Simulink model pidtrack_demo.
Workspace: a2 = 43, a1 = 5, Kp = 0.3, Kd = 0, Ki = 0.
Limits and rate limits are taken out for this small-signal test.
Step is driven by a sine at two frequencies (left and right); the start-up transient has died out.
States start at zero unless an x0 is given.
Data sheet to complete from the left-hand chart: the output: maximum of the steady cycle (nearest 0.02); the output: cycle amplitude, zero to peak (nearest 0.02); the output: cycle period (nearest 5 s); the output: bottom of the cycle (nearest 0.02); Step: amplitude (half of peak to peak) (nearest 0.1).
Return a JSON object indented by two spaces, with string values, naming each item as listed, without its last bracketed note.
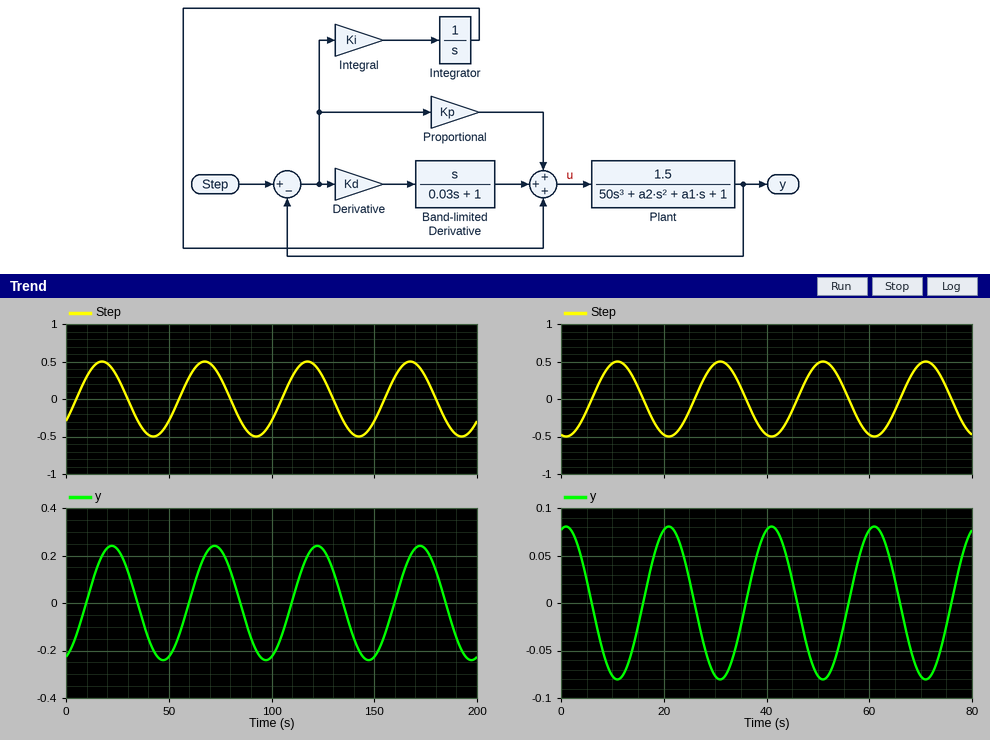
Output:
{
  "the output: maximum of the steady cycle": "0.24",
  "the output: cycle amplitude, zero to peak": "0.24",
  "the output: cycle period": "50 s",
  "the output: bottom of the cycle": "-0.24",
  "Step: amplitude (half of peak to peak)": "0.5"
}
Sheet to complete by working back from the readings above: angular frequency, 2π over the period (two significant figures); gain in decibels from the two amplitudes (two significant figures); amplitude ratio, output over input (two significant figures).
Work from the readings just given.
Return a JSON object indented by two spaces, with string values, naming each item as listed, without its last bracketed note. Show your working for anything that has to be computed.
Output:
{
  "angular frequency, 2π over the period": "2π / 50 = 0.13 rad/s",
  "gain in decibels from the two amplitudes": "20 log10(0.24 / 0.5) = -6.4 dB",
  "amplitude ratio, output over input": "0.24 / 0.5 = 0.48"
}
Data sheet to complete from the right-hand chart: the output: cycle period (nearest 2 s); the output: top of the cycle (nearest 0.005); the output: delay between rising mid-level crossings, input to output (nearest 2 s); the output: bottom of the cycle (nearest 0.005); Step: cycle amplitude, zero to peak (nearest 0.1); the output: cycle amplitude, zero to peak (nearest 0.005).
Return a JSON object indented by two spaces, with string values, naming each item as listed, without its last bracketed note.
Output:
{
  "the output: cycle period": "20 s",
  "the output: top of the cycle": "0.080",
  "the output: delay between rising mid-level crossings, input to output": "10 s",
  "the output: bottom of the cycle": "-0.080",
  "Step: cycle amplitude, zero to peak": "0.5",
  "the output: cycle amplitude, zero to peak": "0.080"
}
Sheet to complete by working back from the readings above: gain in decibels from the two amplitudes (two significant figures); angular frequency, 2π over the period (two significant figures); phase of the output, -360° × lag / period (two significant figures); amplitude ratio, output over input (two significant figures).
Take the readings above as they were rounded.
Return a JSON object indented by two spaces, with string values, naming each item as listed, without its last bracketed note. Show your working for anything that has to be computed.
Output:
{
  "gain in decibels from the two amplitudes": "20 log10(0.08 / 0.5) = -16 dB",
  "angular frequency, 2π over the period": "2π / 20 = 0.31 rad/s",
  "phase of the output, -360° × lag / period": "-360 × 10 / 20 = -180°",
  "amplitude ratio, output over input": "0.08 / 0.5 = 0.16"
}
